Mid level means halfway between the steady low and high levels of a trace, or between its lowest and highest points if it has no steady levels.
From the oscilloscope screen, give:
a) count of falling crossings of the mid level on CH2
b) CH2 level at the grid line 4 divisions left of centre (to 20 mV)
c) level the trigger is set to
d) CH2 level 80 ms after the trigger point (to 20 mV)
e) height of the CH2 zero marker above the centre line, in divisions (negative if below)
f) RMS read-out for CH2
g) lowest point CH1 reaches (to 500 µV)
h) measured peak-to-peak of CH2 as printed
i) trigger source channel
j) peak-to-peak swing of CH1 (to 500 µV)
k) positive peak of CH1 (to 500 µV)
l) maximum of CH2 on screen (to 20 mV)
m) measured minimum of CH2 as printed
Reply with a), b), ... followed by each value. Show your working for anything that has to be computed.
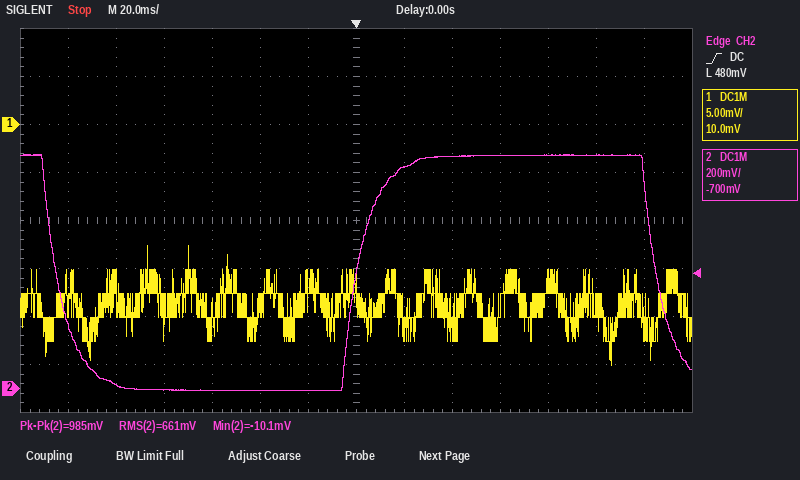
a) 2
b) 0 mV
c) 480 mV
d) 980 mV
e) -3.5 div
f) 661 mV
g) -25.0 mV
h) 985 mV
i) CH2
j) -12.5 mV − (-25.0 mV) = 12.5 mV
k) -12.5 mV
l) 980 mV
m) -10.1 mV
